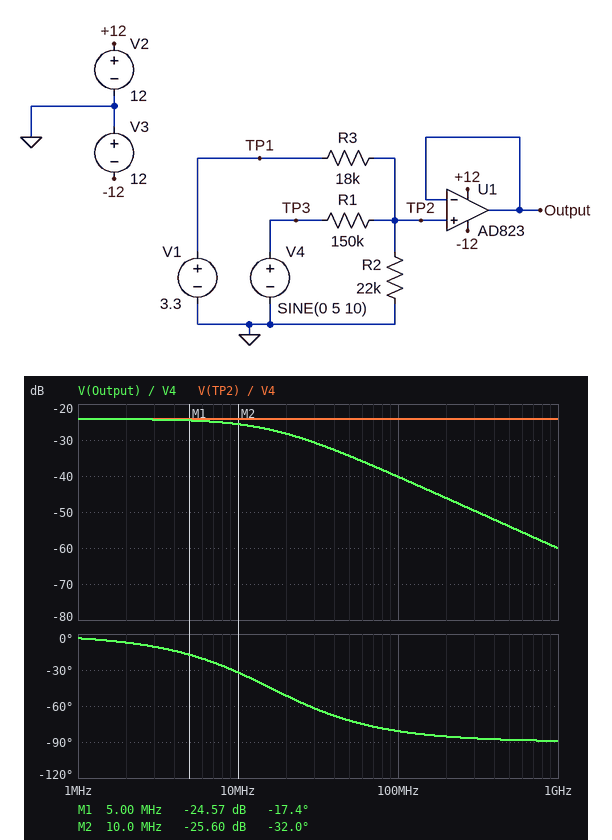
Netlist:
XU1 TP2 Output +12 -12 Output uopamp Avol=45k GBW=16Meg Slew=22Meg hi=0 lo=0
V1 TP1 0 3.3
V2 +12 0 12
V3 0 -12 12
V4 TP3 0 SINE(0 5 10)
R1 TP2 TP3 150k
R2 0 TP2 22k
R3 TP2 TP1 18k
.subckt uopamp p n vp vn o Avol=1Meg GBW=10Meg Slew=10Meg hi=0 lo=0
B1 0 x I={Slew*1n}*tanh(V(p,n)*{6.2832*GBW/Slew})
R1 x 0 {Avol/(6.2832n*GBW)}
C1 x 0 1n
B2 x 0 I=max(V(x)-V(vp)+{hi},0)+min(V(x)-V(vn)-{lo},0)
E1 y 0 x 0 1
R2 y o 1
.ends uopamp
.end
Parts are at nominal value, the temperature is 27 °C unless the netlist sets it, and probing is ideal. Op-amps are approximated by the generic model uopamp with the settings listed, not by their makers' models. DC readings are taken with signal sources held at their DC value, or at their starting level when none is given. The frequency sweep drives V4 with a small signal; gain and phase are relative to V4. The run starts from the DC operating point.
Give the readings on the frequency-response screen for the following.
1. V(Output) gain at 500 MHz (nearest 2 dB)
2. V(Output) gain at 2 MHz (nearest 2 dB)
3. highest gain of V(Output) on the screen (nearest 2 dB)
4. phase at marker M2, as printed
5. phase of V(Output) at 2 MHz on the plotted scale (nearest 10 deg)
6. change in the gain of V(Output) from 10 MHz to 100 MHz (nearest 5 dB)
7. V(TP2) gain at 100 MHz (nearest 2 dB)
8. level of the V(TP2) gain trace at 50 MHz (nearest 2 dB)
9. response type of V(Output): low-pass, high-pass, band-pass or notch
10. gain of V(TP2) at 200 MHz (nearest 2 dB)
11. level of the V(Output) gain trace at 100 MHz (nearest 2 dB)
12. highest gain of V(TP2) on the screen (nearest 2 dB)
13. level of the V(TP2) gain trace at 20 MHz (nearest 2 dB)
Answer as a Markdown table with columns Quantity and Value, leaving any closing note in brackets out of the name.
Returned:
| Quantity | Value |
|---|---|
| V(Output) gain at 500 MHz | -54 dB |
| V(Output) gain at 2 MHz | -24 dB |
| highest gain of V(Output) on the screen | -24 dB |
| phase at marker M2, as printed | -32.0 deg |
| phase of V(Output) at 2 MHz on the plotted scale | -10 deg |
| change in the gain of V(Output) from 10 MHz to 100 MHz | -15 dB |
| V(TP2) gain at 100 MHz | -24 dB |
| level of the V(TP2) gain trace at 50 MHz | -24 dB |
| response type of V(Output): low-pass, high-pass, band-pass or notch | low-pass |
| gain of V(TP2) at 200 MHz | -24 dB |
| level of the V(Output) gain trace at 100 MHz | -40 dB |
| highest gain of V(TP2) on the screen | -24 dB |
| level of the V(TP2) gain trace at 20 MHz | -24 dB |
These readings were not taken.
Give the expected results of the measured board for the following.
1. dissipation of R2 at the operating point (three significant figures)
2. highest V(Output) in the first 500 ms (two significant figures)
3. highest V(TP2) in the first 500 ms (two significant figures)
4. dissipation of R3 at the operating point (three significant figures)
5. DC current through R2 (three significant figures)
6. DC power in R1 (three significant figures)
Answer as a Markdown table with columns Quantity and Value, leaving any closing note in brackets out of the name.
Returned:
| Quantity | Value |
|---|---|
| dissipation of R2 at the operating point | 132 µW |
| highest V(Output) in the first 500 ms | 2.0 V |
| highest V(TP2) in the first 500 ms | 2.0 V |
| dissipation of R3 at the operating point | 142 µW |
| DC current through R2 | 77.4 µA |
| DC power in R1 | 19.3 µW |
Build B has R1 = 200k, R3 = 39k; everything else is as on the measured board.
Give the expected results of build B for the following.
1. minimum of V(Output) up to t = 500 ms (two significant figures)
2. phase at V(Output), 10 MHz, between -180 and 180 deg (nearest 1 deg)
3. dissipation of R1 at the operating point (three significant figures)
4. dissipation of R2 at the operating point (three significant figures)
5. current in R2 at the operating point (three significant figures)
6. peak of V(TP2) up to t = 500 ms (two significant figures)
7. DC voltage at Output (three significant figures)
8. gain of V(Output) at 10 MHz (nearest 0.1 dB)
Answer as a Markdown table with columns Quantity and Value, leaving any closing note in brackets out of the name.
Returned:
| Quantity | Value |
|---|---|
| minimum of V(Output) up to t = 500 ms | 780 mV |
| phase at V(Output), 10 MHz, between -180 and 180 deg | -32 deg |
| dissipation of R1 at the operating point | 6.18 µW |
| dissipation of R2 at the operating point | 56.2 µW |
| current in R2 at the operating point | 50.5 µA |
| peak of V(TP2) up to t = 500 ms | 1.4 V |
| DC voltage at Output | 1.11 V |
| gain of V(Output) at 10 MHz | -25.1 dB |
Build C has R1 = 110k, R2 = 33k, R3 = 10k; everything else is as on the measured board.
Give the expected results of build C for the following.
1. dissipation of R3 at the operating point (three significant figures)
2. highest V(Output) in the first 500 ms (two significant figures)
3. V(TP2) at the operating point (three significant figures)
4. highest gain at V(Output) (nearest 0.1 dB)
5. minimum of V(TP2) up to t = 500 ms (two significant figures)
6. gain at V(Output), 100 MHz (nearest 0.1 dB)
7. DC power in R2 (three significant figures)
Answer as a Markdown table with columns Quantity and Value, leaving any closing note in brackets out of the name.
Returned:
| Quantity | Value |
|---|---|
| dissipation of R3 at the operating point | 87.0 µW |
| highest V(Output) in the first 500 ms | 2.7 V |
| V(TP2) at the operating point | 2.37 V |
| highest gain at V(Output) | -23.7 dB |
| minimum of V(TP2) up to t = 500 ms | 2.0 V |
| gain at V(Output), 100 MHz | -39.7 dB |
| DC power in R2 | 170 µW |
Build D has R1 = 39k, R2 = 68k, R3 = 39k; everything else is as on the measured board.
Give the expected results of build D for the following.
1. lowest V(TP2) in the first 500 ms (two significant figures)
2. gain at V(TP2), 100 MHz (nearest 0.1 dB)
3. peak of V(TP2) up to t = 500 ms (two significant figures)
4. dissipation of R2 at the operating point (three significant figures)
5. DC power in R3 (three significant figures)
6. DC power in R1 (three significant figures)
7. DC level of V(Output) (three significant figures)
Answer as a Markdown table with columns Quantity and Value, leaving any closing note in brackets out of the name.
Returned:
| Quantity | Value |
|---|---|
| lowest V(TP2) in the first 500 ms | -660 mV |
| gain at V(TP2), 100 MHz | -8.2 dB |
| peak of V(TP2) up to t = 500 ms | 3.2 V |
| dissipation of R2 at the operating point | 24.2 µW |
| DC power in R3 | 104 µW |
| DC power in R1 | 42.2 µW |
| DC level of V(Output) | 1.28 V |
